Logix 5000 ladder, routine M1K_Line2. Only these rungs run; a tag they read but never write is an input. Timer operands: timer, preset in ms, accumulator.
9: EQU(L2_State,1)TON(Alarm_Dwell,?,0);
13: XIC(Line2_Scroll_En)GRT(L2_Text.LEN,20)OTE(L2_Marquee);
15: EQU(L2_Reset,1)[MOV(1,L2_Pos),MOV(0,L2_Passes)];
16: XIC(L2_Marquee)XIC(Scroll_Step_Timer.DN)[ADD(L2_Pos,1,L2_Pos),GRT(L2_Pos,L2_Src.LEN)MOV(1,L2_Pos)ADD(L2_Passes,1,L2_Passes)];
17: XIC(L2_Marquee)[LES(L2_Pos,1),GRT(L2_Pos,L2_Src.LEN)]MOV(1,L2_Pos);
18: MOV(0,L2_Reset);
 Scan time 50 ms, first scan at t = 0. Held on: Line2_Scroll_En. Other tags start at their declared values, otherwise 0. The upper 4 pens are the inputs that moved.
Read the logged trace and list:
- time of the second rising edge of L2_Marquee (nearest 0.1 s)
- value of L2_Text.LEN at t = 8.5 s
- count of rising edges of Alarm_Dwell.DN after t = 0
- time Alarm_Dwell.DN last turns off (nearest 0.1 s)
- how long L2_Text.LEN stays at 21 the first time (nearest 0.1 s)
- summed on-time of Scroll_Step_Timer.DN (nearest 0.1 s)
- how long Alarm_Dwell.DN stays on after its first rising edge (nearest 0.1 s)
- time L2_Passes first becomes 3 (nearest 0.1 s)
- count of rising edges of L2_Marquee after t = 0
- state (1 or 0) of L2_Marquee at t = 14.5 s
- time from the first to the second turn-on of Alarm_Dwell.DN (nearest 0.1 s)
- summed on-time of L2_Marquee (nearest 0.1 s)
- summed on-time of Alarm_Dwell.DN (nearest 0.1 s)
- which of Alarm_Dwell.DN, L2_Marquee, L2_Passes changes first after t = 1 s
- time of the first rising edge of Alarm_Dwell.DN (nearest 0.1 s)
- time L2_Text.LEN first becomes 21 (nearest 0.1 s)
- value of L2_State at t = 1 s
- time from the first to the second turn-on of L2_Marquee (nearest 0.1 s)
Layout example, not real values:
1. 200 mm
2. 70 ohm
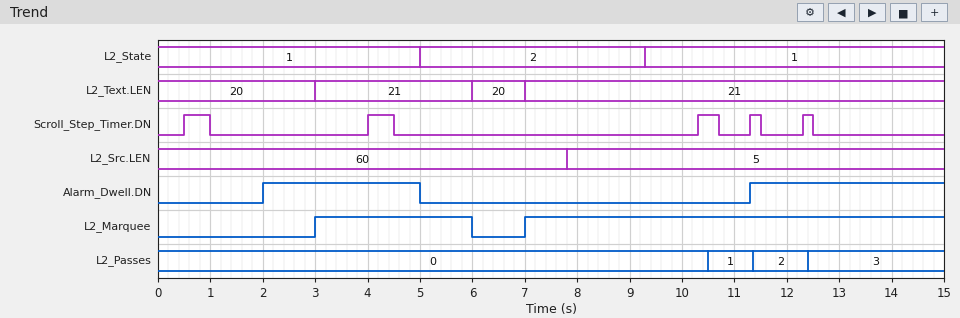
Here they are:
1. 7.0 s
2. 21
3. 2
4. 5.0 s
5. 3.0 s
6. 1.8 s
7. 3.0 s
8. 12.4 s
9. 2
10. 1
11. 9.3 s
12. 11.0 s
13. 6.7 s
14. Alarm_Dwell.DN
15. 2.0 s
16. 3.0 s
17. 1
18. 4.0 s
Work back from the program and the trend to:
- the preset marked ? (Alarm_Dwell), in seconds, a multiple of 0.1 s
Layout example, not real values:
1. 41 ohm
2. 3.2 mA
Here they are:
1. 2.0 s
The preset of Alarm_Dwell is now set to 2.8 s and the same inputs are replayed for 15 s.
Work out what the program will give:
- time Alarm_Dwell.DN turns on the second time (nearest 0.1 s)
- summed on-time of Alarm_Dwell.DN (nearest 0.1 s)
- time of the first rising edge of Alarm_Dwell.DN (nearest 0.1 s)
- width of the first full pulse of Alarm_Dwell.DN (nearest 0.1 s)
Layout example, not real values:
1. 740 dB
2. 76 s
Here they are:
1. 12.1 s
2. 5.1 s
3. 2.8 s
4. 2.2 s
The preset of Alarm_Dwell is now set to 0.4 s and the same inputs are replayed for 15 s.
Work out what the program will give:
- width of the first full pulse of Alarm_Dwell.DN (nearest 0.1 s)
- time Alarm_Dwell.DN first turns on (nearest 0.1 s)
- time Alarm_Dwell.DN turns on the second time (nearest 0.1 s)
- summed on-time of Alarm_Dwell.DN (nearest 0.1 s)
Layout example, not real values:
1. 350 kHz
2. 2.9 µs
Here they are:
1. 4.6 s
2. 0.4 s
3. 9.7 s
4. 9.9 s
